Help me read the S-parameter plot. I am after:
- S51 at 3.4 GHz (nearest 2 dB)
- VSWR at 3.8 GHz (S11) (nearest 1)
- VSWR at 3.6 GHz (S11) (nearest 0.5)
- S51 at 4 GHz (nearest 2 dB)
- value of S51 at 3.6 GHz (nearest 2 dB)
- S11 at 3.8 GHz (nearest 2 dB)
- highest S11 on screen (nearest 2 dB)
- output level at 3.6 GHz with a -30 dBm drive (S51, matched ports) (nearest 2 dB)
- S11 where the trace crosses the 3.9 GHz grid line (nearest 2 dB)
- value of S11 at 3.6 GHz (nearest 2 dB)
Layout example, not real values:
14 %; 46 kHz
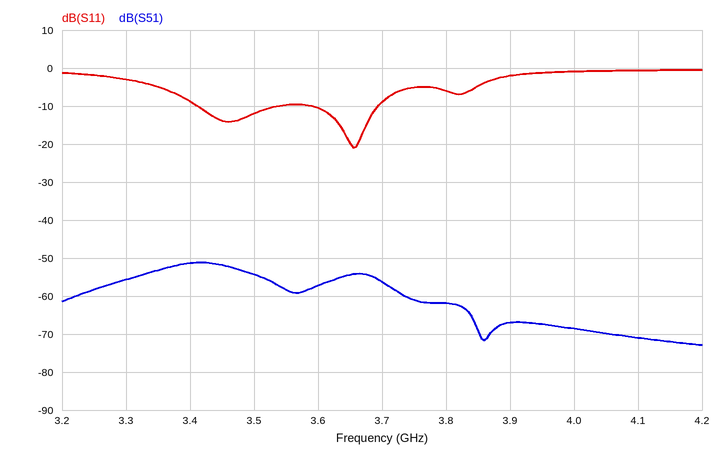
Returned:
-52 dB; 3; 2.0; -68 dB; -58 dB; -6 dB; 0 dB; -88 dBm; -2 dB; -10 dB
